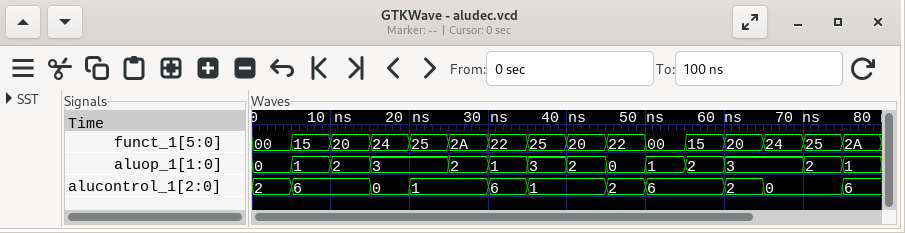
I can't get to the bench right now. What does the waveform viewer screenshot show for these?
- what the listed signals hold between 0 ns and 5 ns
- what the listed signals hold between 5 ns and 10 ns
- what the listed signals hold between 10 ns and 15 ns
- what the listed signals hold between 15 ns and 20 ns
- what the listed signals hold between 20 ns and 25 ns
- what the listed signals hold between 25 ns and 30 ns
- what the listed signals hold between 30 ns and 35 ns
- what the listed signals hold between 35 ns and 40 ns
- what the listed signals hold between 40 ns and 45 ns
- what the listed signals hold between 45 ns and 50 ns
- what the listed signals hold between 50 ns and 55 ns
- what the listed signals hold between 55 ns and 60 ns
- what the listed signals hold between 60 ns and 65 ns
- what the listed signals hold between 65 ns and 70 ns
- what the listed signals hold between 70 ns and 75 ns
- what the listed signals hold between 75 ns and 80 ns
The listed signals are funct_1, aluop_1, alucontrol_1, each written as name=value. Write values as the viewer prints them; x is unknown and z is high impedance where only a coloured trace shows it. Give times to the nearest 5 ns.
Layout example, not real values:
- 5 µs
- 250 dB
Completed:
- funct_1=00, aluop_1=0, alucontrol_1=2
- funct_1=15, aluop_1=1, alucontrol_1=6
- funct_1=20, aluop_1=2, alucontrol_1=6
- funct_1=24, aluop_1=3, alucontrol_1=0
- funct_1=25, aluop_1=3, alucontrol_1=1
- funct_1=2A, aluop_1=2, alucontrol_1=1
- funct_1=22, aluop_1=1, alucontrol_1=6
- funct_1=25, aluop_1=3, alucontrol_1=1
- funct_1=20, aluop_1=2, alucontrol_1=1
- funct_1=22, aluop_1=0, alucontrol_1=2
- funct_1=00, aluop_1=1, alucontrol_1=6
- funct_1=15, aluop_1=2, alucontrol_1=6
- funct_1=20, aluop_1=3, alucontrol_1=2
- funct_1=24, aluop_1=3, alucontrol_1=0
- funct_1=25, aluop_1=2, alucontrol_1=0
- funct_1=2A, aluop_1=1, alucontrol_1=6
